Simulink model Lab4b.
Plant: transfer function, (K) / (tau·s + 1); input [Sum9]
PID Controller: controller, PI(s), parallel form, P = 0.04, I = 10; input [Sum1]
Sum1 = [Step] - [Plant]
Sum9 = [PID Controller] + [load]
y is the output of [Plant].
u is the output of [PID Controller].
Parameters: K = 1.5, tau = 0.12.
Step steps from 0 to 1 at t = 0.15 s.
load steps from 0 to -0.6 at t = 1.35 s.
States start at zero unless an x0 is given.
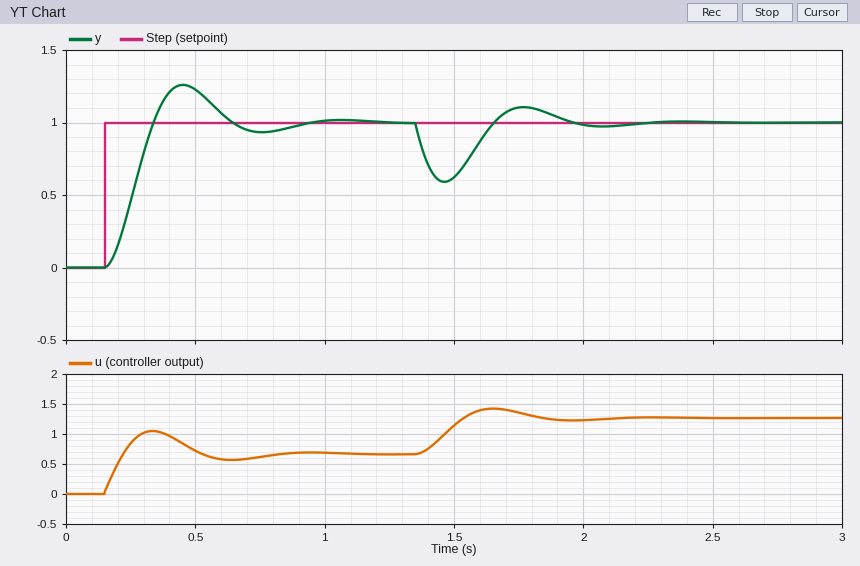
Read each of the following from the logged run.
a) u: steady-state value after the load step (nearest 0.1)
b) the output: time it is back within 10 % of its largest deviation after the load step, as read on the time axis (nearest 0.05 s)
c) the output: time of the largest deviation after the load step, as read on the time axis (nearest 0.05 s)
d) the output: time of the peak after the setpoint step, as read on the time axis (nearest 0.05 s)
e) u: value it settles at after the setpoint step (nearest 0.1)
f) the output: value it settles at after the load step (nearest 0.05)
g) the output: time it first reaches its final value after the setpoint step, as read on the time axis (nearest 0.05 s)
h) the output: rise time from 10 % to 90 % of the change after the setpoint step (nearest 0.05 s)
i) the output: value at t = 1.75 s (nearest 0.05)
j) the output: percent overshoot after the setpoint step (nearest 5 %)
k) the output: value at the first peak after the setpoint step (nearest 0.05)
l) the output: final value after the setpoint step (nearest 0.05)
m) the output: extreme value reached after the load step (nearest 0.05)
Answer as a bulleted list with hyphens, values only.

- 1.3
- 1.90 s
- 1.45 s
- 0.45 s
- 0.7
- 1.00
- 0.35 s
- 0.15 s
- 1.10
- 25 %
- 1.25
- 1.00
- 0.60
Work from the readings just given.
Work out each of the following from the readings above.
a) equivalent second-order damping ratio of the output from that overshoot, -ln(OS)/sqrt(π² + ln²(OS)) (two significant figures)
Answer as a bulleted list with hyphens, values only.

- 0.40
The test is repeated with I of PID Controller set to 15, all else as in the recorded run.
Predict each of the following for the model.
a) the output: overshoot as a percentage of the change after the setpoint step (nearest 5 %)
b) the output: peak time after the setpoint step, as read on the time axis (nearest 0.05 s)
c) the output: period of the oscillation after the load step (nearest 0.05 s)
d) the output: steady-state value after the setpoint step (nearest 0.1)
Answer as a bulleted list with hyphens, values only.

- 35 %
- 0.40 s
- 0.50 s
- 1.0
